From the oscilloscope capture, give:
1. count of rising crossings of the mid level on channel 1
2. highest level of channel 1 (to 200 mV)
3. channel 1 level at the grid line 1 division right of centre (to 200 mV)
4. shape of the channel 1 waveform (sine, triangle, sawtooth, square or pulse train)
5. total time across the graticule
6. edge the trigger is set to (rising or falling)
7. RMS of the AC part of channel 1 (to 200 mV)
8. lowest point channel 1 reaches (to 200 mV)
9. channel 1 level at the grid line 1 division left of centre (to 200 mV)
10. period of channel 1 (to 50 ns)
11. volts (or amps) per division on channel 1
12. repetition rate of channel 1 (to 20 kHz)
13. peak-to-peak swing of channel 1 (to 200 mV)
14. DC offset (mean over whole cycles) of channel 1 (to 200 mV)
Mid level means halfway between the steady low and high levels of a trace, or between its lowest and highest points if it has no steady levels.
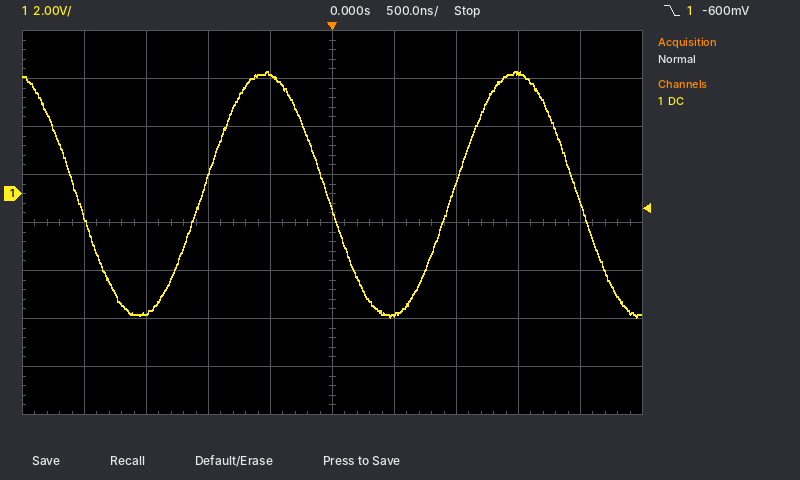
2
5.0 V
-5.0 V
sine
5 µs
falling
3.6 V
-5.2 V
5.0 V
2.00 µs
2 V
500 kHz
10.2 V
0.0 V
